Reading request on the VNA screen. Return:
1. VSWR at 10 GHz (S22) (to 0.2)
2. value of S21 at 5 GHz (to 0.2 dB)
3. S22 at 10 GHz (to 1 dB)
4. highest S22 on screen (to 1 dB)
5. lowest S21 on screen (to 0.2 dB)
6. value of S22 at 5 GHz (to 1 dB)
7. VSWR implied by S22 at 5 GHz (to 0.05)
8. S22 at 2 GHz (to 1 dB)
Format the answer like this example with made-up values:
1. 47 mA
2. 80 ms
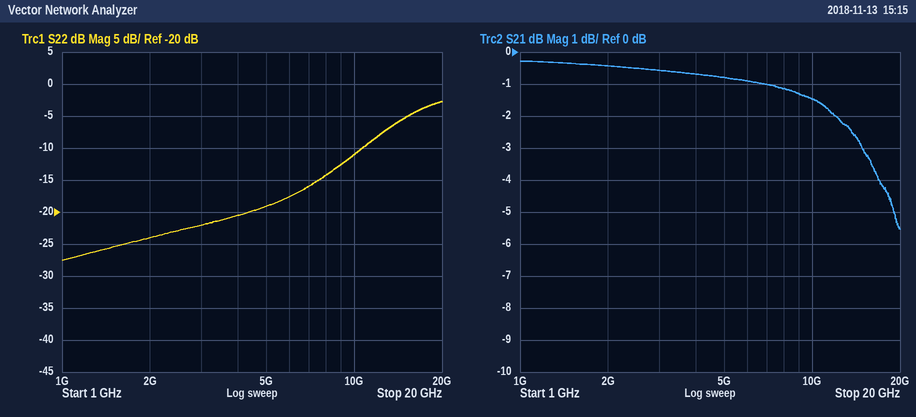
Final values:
1. 1.8
2. -0.8 dB
3. -11 dB
4. -3 dB
5. -5.6 dB
6. -19 dB
7. 1.25
8. -24 dB
